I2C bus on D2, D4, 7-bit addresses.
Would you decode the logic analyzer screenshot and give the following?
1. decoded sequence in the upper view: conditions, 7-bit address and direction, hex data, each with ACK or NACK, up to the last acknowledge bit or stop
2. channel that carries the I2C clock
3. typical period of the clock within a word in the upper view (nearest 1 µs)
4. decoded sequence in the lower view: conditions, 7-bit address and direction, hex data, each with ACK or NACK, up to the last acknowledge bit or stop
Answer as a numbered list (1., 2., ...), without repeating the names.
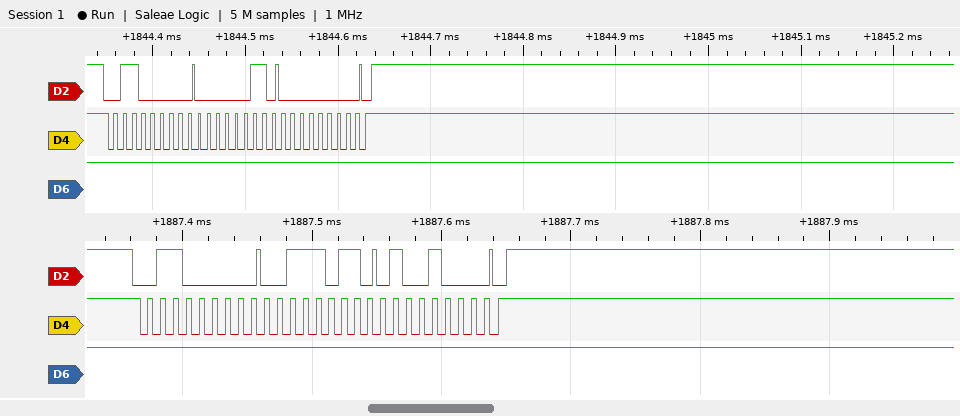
1. start, address 30 write ACK, 03 ACK, 00 ACK, stop
2. D4
3. 10 µs
4. start, address 30 write ACK, 3B ACK, 48 ACK, stop
